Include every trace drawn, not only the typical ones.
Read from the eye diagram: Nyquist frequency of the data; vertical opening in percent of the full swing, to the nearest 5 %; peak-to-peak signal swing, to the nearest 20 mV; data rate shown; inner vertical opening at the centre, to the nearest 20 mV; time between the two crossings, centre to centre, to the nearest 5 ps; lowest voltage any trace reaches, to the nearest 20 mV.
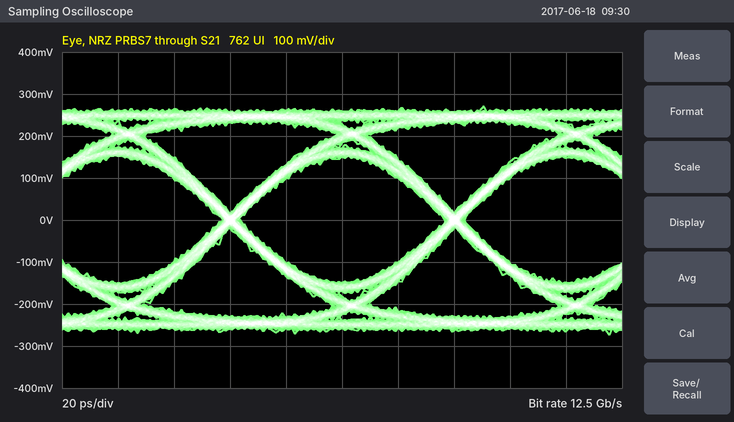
6.25 GHz
55 %
540 mV
12.5 Gb/s
300 mV
80 ps
-280 mV
